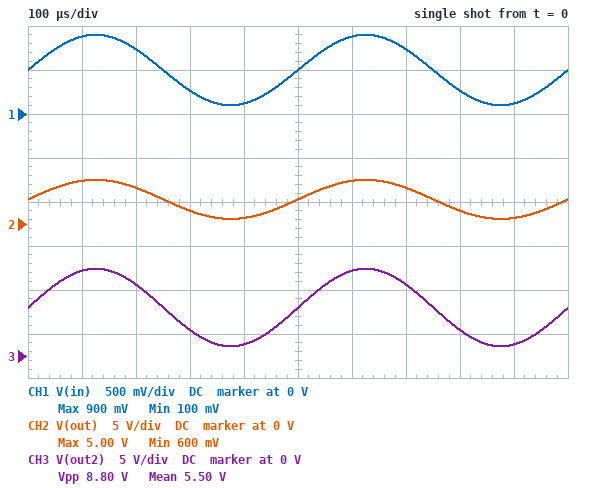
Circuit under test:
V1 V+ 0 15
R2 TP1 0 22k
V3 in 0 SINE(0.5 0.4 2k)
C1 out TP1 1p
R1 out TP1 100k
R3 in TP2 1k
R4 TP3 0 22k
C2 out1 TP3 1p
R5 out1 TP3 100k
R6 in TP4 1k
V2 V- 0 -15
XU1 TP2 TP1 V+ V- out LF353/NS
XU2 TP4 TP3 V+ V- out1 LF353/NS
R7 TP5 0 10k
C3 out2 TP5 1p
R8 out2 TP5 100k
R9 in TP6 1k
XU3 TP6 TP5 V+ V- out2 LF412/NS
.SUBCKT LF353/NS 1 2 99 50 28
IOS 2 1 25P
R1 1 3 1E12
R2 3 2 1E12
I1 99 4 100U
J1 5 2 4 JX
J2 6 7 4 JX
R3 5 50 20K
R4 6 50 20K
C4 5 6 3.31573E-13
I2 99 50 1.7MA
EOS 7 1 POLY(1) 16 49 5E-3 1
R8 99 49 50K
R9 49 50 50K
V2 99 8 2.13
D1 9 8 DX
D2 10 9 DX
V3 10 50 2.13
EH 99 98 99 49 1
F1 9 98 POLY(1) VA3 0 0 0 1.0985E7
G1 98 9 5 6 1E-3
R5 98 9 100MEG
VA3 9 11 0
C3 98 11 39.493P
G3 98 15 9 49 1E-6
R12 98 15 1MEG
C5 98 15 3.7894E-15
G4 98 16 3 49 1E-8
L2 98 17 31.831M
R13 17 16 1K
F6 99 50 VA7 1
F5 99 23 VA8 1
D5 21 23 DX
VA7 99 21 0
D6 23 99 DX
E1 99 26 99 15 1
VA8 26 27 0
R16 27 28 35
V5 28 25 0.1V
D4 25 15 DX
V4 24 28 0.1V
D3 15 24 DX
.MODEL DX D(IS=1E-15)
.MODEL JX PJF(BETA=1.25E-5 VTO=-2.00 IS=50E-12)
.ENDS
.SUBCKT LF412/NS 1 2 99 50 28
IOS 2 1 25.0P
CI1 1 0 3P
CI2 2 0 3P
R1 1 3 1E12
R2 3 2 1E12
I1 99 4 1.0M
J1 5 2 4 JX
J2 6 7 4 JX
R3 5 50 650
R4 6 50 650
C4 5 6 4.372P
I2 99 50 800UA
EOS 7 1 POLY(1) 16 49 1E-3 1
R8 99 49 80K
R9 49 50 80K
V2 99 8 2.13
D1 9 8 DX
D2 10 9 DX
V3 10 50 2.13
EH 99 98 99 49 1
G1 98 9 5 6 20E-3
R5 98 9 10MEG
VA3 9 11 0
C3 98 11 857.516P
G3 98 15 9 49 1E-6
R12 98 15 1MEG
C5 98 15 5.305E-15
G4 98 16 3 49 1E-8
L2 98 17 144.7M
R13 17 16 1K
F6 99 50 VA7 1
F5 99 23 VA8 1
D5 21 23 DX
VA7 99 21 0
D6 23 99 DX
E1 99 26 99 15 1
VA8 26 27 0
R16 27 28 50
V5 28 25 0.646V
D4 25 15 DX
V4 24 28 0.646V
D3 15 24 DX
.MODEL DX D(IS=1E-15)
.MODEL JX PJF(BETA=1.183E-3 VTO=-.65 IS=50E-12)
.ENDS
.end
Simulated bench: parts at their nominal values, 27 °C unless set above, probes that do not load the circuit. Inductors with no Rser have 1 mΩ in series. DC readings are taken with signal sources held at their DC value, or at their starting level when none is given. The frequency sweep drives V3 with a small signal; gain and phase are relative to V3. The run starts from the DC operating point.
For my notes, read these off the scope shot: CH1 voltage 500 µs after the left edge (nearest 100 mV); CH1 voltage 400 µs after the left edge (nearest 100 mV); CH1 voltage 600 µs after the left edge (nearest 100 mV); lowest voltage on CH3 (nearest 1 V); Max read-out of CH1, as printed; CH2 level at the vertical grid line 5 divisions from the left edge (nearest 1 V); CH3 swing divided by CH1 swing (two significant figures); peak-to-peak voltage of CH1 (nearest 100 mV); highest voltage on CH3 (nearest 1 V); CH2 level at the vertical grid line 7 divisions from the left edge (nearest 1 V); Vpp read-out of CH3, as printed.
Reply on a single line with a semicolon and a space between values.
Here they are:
500 mV; 100 mV; 900 mV; 1 V; 900 mV; 3 V; 11; 800 mV; 10 V; 4 V; 8.80 V
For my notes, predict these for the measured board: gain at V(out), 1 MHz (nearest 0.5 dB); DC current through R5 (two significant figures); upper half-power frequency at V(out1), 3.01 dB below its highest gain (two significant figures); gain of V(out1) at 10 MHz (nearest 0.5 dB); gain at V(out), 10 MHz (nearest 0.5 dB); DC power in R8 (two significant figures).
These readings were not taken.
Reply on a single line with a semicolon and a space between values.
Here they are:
8.5 dB; 23 µA; 540 kHz; -10.0 dB; -10.0 dB; 250 µW
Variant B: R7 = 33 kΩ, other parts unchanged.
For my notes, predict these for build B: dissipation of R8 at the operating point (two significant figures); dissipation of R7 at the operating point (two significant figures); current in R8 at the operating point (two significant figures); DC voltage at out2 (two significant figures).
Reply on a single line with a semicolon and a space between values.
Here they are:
23 µW; 7.6 µW; 15 µA; 2.0 V
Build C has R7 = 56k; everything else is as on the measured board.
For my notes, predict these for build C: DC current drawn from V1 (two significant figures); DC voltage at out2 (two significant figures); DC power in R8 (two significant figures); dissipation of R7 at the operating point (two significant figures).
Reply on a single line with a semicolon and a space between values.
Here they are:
6.2 mA; 1.4 V; 8.0 µW; 4.5 µW
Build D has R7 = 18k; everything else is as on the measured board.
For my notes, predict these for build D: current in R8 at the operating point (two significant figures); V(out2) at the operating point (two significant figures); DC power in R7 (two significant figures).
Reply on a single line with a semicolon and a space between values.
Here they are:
28 µA; 3.3 V; 14 µW
